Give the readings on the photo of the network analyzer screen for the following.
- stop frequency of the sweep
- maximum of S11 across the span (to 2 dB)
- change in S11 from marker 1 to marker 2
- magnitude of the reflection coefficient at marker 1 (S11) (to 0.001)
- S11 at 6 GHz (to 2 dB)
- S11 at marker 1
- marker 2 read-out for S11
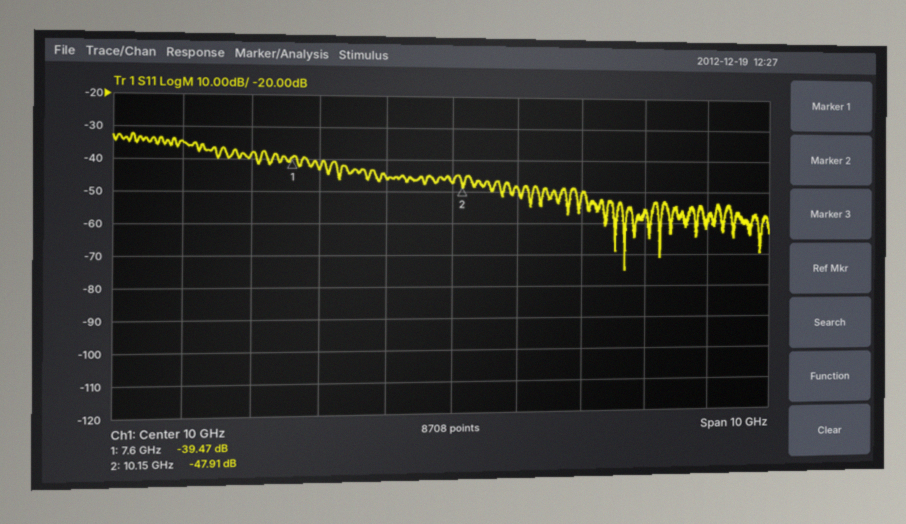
15 GHz
-32 dB
-8.44 dB
0.011
-34 dB
-39.47 dB
-47.91 dB
